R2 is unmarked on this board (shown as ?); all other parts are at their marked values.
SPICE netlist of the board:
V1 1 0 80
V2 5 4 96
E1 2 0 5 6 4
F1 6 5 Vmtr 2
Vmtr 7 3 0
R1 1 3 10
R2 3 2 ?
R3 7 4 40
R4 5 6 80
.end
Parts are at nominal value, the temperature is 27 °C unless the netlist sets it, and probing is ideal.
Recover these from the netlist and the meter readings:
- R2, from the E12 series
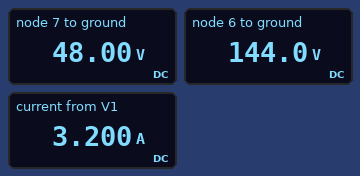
15 Ω
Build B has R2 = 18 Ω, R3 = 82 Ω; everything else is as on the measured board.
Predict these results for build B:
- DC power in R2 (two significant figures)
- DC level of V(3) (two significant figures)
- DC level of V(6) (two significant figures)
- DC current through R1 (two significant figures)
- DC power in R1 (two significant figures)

150 W
51 V
150 V
2.9 A
82 W
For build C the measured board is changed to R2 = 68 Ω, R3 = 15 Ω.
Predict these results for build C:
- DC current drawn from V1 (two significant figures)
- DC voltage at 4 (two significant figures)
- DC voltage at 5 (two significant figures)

1.0 A
70 V
170 V
